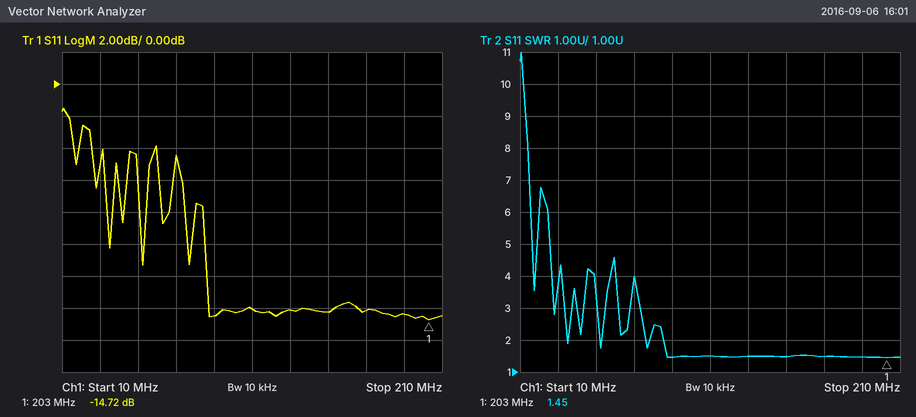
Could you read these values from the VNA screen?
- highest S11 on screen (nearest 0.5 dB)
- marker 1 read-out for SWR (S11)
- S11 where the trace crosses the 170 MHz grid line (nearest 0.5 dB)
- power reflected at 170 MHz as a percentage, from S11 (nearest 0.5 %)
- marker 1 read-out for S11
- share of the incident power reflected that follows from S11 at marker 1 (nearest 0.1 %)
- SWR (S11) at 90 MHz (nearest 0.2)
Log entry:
-1.5 dB
1.45
-14.0 dB
4.0 %
-14.72 dB
3.4 %
1.4
